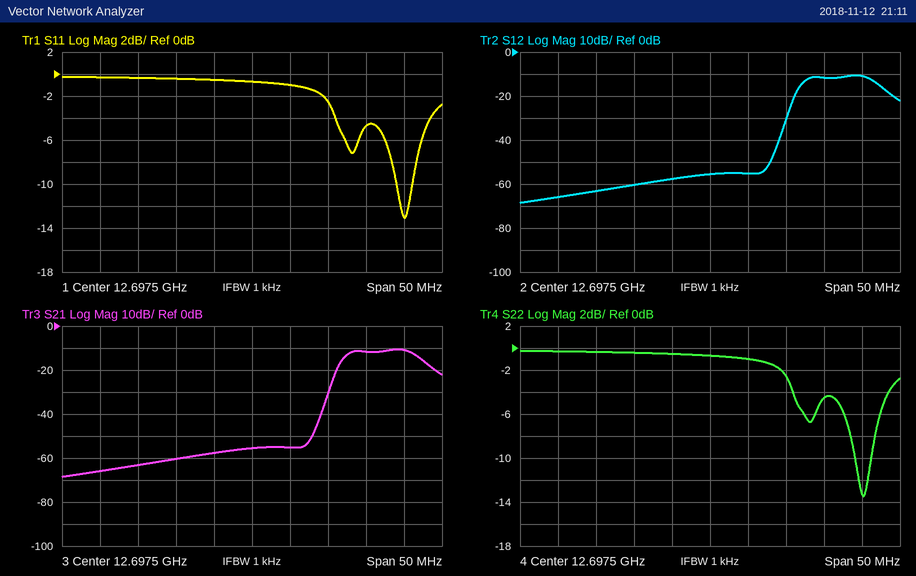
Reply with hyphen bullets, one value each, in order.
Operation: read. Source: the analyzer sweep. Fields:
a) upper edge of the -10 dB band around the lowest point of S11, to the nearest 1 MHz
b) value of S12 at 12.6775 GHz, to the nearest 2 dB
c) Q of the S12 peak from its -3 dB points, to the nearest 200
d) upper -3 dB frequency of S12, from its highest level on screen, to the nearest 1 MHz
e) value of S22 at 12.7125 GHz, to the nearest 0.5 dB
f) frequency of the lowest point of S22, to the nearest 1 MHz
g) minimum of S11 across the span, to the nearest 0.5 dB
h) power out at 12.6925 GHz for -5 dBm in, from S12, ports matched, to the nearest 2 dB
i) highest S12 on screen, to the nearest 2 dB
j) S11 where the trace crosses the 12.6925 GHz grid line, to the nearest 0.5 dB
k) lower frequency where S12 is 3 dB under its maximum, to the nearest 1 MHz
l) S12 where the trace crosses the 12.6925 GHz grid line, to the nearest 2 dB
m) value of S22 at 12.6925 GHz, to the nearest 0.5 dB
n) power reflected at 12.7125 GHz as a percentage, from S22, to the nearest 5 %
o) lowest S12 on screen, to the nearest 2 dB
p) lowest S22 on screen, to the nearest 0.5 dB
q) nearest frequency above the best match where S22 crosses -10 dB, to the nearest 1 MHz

- 12.719 GHz
- -66 dB
- 1400
- 12.719 GHz
- -4.5 dB
- 12.718 GHz
- -13.0 dB
- -62 dBm
- -10 dB
- -0.5 dB
- 12.710 GHz
- -58 dB
- -0.5 dB
- 35 %
- -68 dB
- -13.5 dB
- 12.719 GHz
